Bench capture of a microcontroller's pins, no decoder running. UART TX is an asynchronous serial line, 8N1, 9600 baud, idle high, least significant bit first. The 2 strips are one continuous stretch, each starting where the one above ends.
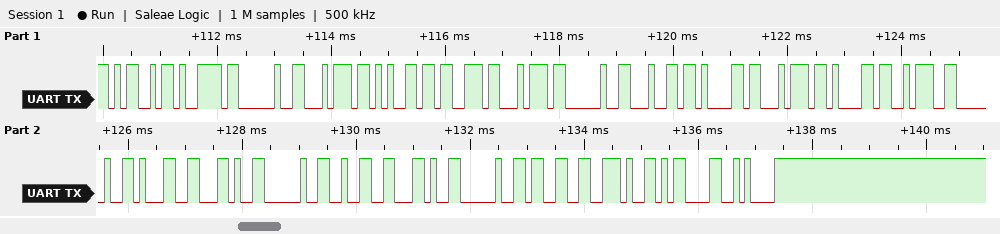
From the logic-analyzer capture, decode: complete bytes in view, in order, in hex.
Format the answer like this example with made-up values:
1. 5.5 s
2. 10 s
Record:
1. 4D 79 20 74 65 73 74 20 64 61 74 61 3A 20 31 2C 20 32 2C 20 33 2E 0D 0A
